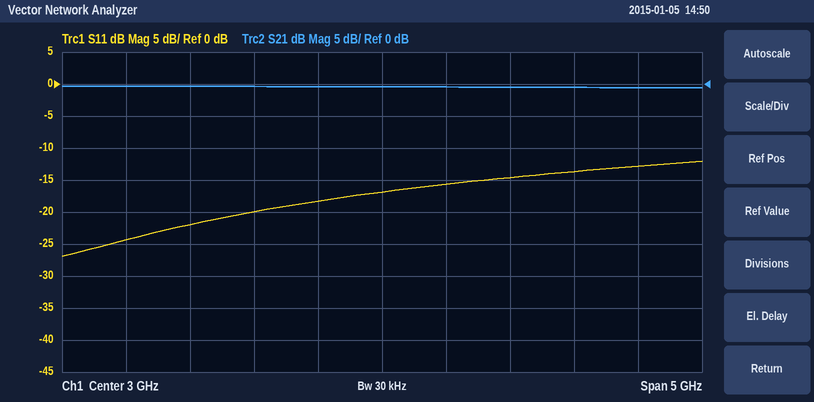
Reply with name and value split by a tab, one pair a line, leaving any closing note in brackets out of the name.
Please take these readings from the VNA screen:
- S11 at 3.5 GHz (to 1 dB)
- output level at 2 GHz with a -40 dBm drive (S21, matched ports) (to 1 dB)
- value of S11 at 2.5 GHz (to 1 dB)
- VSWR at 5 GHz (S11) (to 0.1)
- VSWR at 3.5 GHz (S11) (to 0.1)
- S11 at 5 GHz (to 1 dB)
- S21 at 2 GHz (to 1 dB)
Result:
S11 at 3.5 GHz	-16 dB
output level at 2 GHz with a -40 dBm drive (S21, matched ports)	-40 dBm
value of S11 at 2.5 GHz	-18 dB
VSWR at 5 GHz (S11)	1.6
VSWR at 3.5 GHz (S11)	1.4
S11 at 5 GHz	-13 dB
S21 at 2 GHz	0 dB
